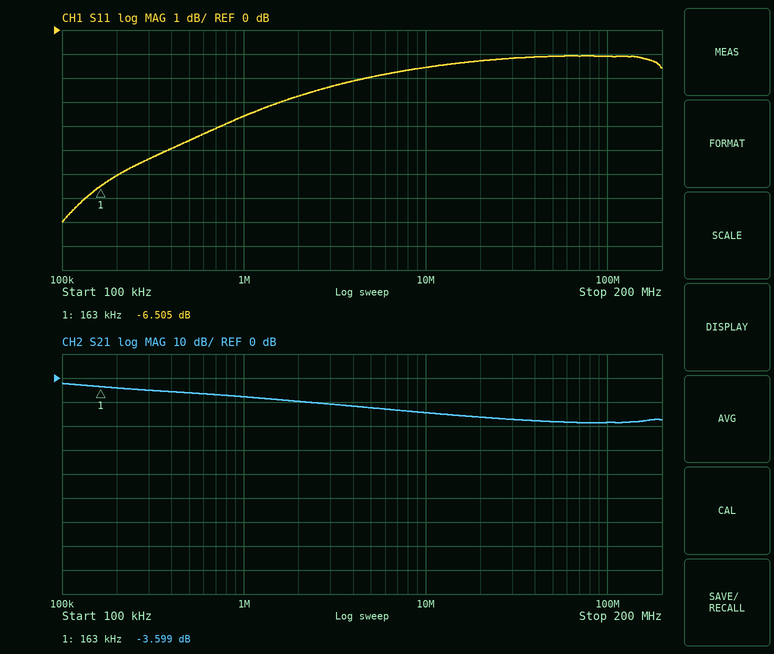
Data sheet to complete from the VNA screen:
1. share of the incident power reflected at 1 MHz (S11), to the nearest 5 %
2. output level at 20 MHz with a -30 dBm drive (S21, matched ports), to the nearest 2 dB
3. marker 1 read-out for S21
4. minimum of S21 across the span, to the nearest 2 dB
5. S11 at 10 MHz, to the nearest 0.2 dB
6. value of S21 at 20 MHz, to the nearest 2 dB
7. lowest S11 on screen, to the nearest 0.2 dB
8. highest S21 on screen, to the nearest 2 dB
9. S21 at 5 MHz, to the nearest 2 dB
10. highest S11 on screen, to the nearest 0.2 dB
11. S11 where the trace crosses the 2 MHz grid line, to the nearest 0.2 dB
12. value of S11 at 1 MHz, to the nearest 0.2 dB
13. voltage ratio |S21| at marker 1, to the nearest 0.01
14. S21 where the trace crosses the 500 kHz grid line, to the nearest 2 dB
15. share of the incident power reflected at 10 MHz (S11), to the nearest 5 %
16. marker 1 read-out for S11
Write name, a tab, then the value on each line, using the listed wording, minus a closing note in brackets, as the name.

share of the incident power reflected at 1 MHz (S11), to the nearest 5 %	45 %
output level at 20 MHz with a -30 dBm drive (S21, matched ports), to the nearest 2 dB	-46 dBm
marker 1 read-out for S21	-3.599 dB
minimum of S21 across the span, to the nearest 2 dB	-18 dB
S11 at 10 MHz, to the nearest 0.2 dB	-1.6 dB
value of S21 at 20 MHz, to the nearest 2 dB	-16 dB
lowest S11 on screen, to the nearest 0.2 dB	-8.0 dB
highest S21 on screen, to the nearest 2 dB	-2 dB
S21 at 5 MHz, to the nearest 2 dB	-12 dB
highest S11 on screen, to the nearest 0.2 dB	-1.0 dB
S11 where the trace crosses the 2 MHz grid line, to the nearest 0.2 dB	-2.8 dB
value of S11 at 1 MHz, to the nearest 0.2 dB	-3.6 dB
voltage ratio |S21| at marker 1, to the nearest 0.01	0.66
S21 where the trace crosses the 500 kHz grid line, to the nearest 2 dB	-6 dB
share of the incident power reflected at 10 MHz (S11), to the nearest 5 %	70 %
marker 1 read-out for S11	-6.505 dB
